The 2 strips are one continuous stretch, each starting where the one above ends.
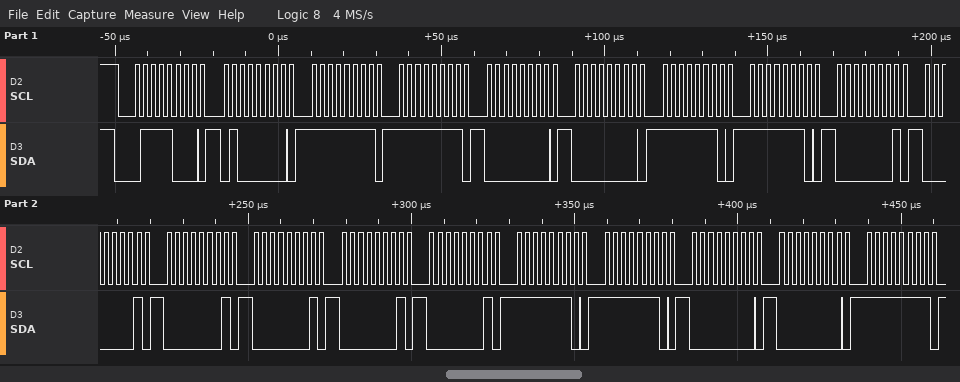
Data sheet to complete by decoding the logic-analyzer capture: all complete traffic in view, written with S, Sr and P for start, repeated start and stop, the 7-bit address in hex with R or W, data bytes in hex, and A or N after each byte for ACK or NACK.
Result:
S 3CW A 40 A FF A FF A 00 A 00 A FE A FE A 01 A 01 A 01 A 01 A 01 A 01 A FE A FE A 00 A 00 A FF A
